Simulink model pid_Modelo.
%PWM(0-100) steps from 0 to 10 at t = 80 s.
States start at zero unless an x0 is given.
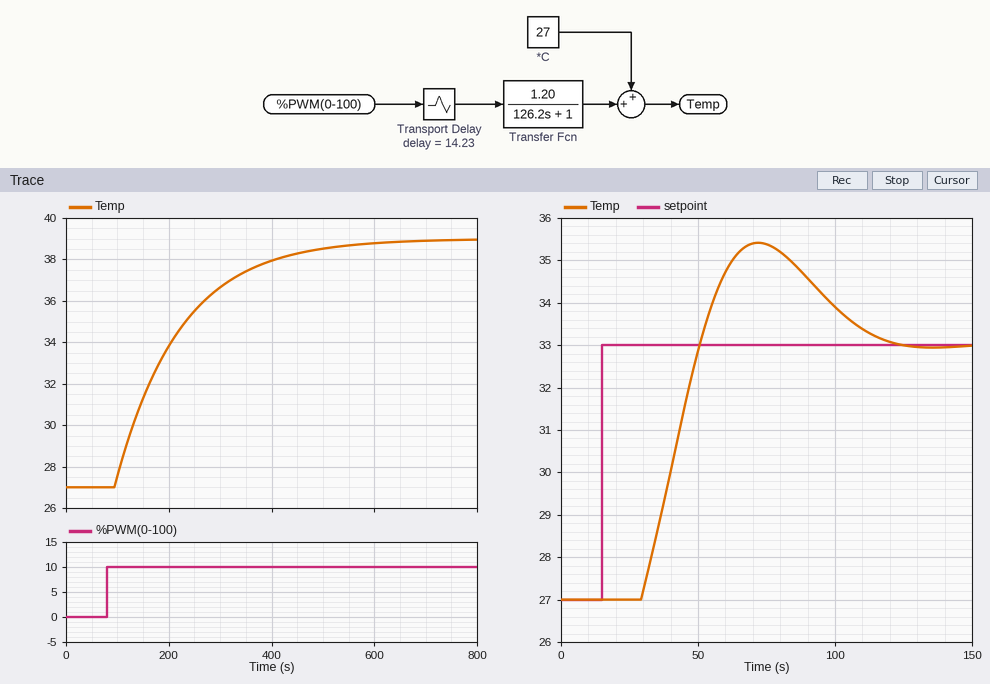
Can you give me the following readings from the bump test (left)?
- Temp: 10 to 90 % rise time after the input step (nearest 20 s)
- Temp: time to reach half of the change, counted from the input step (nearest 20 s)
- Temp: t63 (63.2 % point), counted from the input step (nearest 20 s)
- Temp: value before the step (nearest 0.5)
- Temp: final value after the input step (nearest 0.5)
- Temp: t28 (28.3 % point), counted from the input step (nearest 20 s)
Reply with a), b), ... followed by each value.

a) 280 s
b) 100 s
c) 140 s
d) 27.0
e) 39.0
f) 60 s
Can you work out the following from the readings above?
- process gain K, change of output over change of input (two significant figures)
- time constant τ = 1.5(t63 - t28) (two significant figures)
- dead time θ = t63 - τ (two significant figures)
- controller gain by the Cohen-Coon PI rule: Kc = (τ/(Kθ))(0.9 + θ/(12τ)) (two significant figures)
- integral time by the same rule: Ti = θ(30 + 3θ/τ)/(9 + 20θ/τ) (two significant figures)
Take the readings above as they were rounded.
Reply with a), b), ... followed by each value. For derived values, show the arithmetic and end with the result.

a) (39 - 27) / 10 = 1.2
b) 1.5 × (140 - 60) = 120 s
c) 140 - 120 = 20 s
d) 120 / (1.2 × 20) × (0.9 + 20 / (12 × 120)) = 4.6
e) 20 × (30 + 3 × 20 / 120) / (9 + 20 × 20 / 120) = 49 s
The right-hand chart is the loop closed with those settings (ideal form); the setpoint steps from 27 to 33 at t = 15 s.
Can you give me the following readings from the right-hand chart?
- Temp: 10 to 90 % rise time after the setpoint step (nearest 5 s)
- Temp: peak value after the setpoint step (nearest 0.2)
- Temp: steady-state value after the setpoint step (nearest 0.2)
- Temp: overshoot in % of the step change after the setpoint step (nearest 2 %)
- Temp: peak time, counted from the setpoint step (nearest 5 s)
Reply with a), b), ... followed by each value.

a) 15 s
b) 35.4
c) 33.0
d) 40 %
e) 55 s
